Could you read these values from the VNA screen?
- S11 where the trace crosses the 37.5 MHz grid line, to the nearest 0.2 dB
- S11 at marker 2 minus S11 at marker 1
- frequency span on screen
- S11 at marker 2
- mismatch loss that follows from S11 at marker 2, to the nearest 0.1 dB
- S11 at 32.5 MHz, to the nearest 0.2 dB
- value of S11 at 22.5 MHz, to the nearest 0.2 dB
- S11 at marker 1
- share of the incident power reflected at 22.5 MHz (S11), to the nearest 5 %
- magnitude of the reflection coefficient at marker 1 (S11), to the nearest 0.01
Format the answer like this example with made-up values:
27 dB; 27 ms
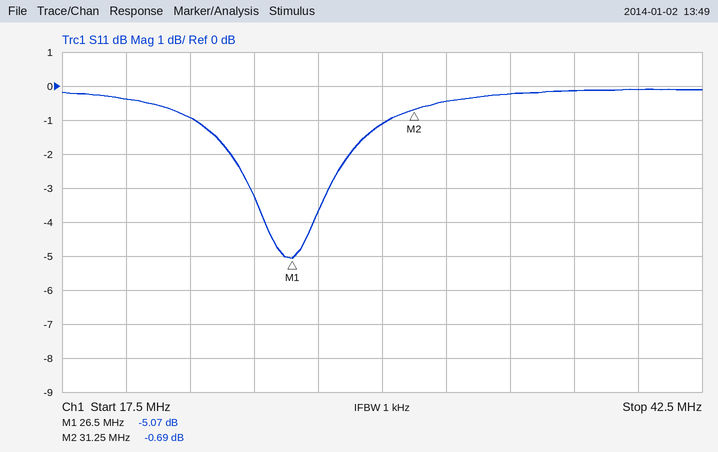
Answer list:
-0.2 dB; 4.38 dB; 25 MHz; -0.69 dB; 8.3 dB; -0.4 dB; -1.0 dB; -5.07 dB; 80 %; 0.56
